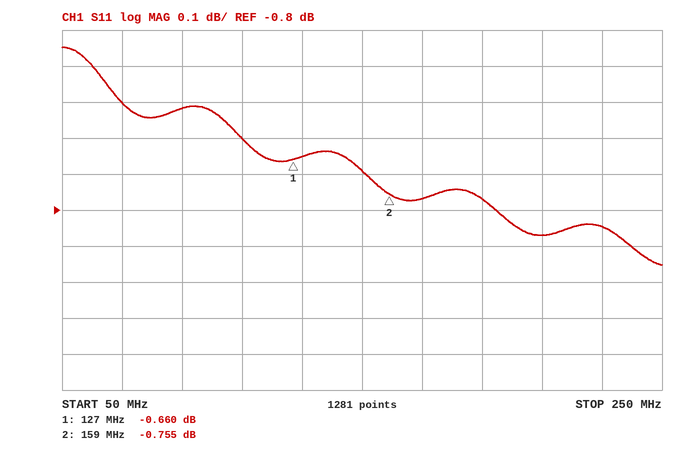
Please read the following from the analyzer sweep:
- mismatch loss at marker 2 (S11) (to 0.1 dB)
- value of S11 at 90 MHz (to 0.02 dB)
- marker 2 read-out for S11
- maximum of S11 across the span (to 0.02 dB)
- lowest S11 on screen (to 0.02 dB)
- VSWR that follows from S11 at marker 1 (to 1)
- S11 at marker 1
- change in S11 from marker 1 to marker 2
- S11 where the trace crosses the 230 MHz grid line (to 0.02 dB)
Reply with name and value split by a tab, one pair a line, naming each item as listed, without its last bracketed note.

mismatch loss at marker 2 (S11)	8.0 dB
value of S11 at 90 MHz	-0.52 dB
marker 2 read-out for S11	-0.755 dB
maximum of S11 across the span	-0.34 dB
lowest S11 on screen	-0.96 dB
VSWR that follows from S11 at marker 1	26
S11 at marker 1	-0.660 dB
change in S11 from marker 1 to marker 2	-0.095 dB
S11 where the trace crosses the 230 MHz grid line	-0.84 dB
